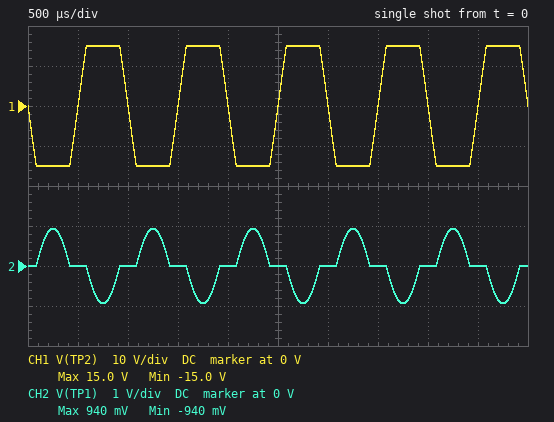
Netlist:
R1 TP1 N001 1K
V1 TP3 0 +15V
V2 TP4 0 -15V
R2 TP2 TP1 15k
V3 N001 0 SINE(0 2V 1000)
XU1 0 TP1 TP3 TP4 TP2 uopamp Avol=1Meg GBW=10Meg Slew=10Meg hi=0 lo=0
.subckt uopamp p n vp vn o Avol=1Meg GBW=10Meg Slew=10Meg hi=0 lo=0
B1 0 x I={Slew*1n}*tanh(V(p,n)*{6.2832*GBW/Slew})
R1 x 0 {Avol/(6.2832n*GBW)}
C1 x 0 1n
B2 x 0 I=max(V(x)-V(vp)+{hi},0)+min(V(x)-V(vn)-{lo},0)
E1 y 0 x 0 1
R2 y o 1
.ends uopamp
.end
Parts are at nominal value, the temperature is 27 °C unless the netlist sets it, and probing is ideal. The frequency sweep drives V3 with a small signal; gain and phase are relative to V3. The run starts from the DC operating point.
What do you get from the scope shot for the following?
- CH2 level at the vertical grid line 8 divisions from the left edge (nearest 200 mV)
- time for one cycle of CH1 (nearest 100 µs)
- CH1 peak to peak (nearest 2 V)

0 V
1.0 ms
30 V
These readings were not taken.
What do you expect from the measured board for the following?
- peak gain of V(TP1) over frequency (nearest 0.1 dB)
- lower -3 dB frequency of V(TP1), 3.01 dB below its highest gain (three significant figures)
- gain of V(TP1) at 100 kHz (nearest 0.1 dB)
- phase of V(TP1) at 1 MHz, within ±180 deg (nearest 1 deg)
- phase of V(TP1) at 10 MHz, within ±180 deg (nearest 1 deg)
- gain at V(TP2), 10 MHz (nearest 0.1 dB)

-0.6 dB
625 kHz
-16.6 dB
32 deg
4 deg
-0.6 dB
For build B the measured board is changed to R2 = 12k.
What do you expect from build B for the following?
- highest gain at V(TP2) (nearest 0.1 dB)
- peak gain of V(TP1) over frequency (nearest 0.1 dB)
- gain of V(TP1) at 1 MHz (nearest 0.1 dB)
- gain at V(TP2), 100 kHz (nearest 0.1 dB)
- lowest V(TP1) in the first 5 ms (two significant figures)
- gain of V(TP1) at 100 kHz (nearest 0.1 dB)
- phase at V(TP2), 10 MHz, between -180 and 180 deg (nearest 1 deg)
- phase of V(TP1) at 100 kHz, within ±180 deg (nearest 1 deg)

21.6 dB
-0.7 dB
-2.7 dB
21.5 dB
-690 mV
-18.5 dB
94 deg
83 deg
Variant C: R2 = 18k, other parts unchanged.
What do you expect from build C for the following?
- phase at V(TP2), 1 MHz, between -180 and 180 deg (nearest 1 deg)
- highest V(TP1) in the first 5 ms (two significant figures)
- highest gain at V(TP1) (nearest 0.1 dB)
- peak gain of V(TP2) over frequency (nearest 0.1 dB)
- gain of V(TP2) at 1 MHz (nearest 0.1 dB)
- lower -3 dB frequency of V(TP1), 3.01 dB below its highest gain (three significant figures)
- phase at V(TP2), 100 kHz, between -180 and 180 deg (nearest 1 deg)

118 deg
1.1 V
-0.5 dB
25.1 dB
18.5 dB
526 kHz
169 deg
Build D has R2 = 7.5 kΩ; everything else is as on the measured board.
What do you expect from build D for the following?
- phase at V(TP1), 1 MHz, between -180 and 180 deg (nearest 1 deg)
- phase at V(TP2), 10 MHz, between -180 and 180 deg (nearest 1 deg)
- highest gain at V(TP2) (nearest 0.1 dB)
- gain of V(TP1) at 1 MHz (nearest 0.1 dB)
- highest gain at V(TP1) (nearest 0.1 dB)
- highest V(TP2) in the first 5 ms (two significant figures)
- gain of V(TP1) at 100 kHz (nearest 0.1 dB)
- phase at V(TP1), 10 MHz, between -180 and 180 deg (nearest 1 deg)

50 deg
97 deg
17.5 dB
-4.9 dB
-1.1 dB
15 V
-22.5 dB
7 deg
